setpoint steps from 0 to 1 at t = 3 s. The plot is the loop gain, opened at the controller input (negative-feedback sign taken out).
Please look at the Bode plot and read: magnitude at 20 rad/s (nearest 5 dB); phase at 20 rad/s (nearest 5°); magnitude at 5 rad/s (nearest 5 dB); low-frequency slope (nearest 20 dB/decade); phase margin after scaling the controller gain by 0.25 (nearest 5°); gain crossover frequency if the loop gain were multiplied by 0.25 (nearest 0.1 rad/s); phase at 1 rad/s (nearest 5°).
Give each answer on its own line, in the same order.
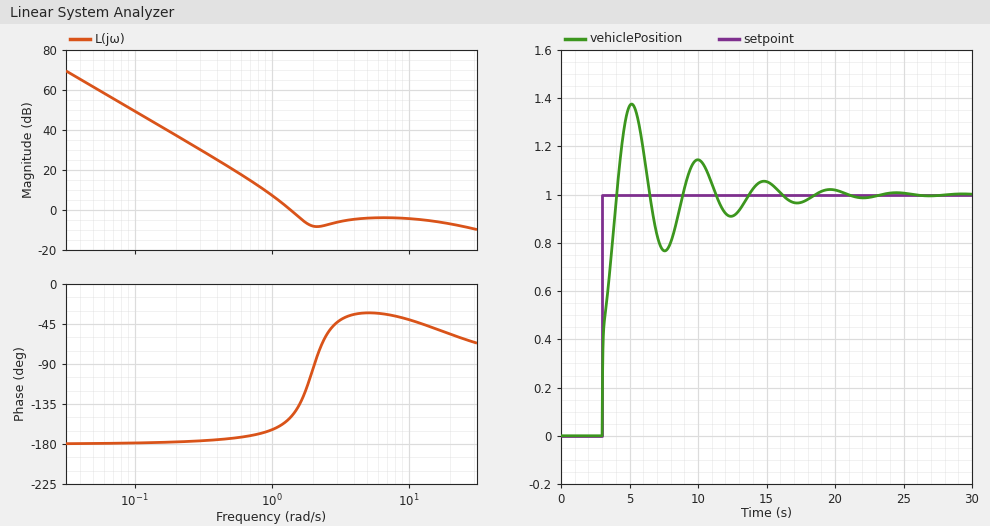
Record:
-5 dB
-55°
-5 dB
-40 dB/decade
10°
0.8 rad/s
-165°
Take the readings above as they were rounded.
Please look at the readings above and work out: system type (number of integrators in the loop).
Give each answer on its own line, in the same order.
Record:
2
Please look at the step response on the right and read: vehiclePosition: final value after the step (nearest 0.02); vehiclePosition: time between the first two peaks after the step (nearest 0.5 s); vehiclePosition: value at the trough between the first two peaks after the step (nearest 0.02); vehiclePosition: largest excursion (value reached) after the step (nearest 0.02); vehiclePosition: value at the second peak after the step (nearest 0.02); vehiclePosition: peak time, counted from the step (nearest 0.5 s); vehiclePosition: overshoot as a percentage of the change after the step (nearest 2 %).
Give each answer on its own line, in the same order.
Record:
1.00
5.0 s
0.76
1.38
1.14
2.0 s
38 %
